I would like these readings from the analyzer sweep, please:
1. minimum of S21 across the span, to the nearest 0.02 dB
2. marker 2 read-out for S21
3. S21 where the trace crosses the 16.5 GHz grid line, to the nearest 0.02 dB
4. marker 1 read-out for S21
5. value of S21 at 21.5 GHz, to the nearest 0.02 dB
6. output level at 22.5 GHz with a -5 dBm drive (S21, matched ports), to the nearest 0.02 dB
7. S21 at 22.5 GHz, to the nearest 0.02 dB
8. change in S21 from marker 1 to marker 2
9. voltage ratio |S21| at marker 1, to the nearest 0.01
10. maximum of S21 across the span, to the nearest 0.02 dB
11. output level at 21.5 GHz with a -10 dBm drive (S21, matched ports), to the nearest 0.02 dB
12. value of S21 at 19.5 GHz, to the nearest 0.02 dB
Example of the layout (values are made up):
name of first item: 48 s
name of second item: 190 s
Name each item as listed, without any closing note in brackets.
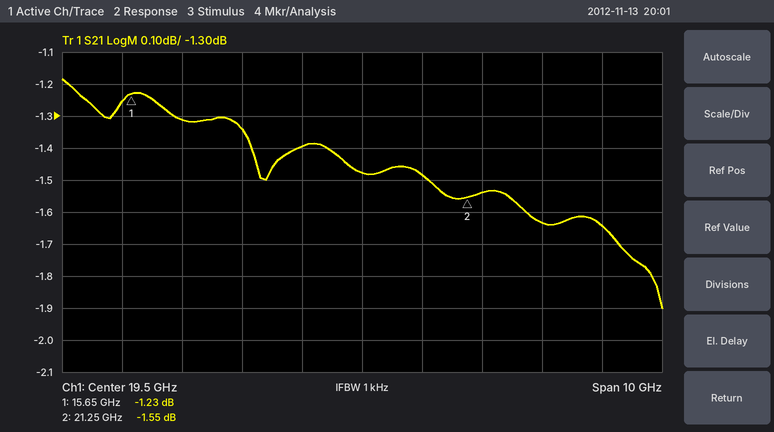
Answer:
minimum of S21 across the span, to the nearest 0.02 dB: -1.90 dB
marker 2 read-out for S21: -1.55 dB
S21 where the trace crosses the 16.5 GHz grid line, to the nearest 0.02 dB: -1.32 dB
marker 1 read-out for S21: -1.23 dB
value of S21 at 21.5 GHz, to the nearest 0.02 dB: -1.54 dB
output level at 22.5 GHz with a -5 dBm drive (S21, matched ports), to the nearest 0.02 dB: -6.64 dBm
S21 at 22.5 GHz, to the nearest 0.02 dB: -1.64 dB
change in S21 from marker 1 to marker 2: -0.32 dB
voltage ratio |S21| at marker 1, to the nearest 0.01: 0.87
maximum of S21 across the span, to the nearest 0.02 dB: -1.18 dB
output level at 21.5 GHz with a -10 dBm drive (S21, matched ports), to the nearest 0.02 dB: -11.54 dBm
value of S21 at 19.5 GHz, to the nearest 0.02 dB: -1.48 dB
